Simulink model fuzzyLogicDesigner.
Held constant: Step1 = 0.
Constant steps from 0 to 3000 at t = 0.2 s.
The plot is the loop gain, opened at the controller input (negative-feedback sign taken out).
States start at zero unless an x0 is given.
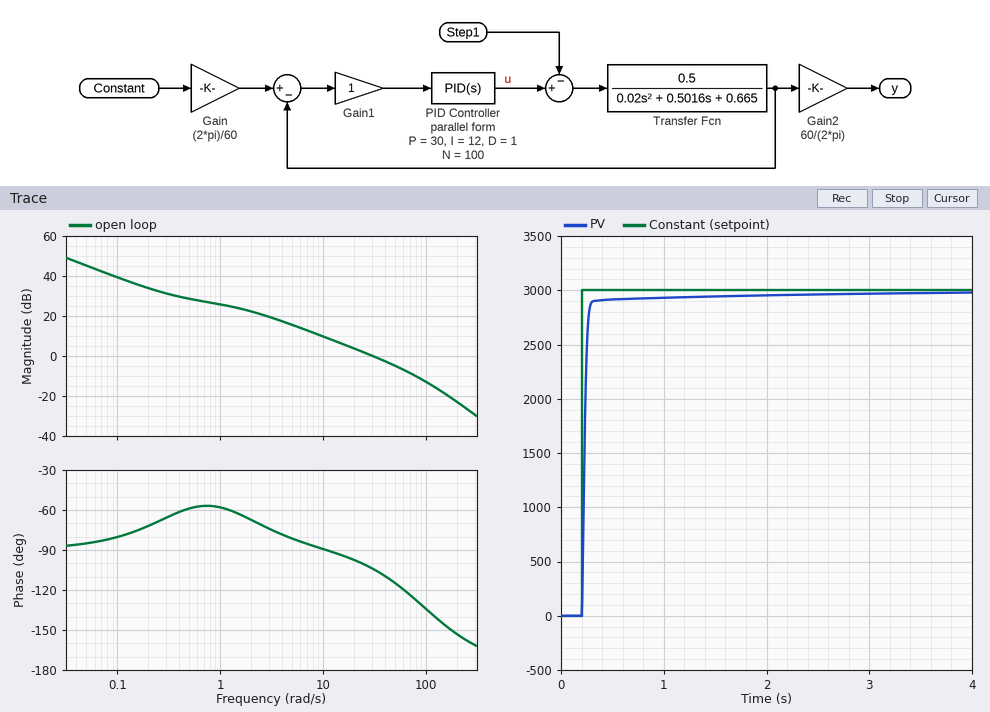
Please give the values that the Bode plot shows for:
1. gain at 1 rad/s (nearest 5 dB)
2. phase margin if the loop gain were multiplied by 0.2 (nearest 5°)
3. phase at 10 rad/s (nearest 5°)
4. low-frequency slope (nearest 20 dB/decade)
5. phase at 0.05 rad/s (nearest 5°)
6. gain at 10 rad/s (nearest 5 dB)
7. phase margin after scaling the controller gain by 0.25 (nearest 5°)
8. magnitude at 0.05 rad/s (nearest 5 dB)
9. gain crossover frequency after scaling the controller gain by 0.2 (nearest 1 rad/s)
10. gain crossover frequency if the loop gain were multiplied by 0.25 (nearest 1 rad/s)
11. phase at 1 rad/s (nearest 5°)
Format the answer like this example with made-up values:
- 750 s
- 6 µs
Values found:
- 25 dB
- 95°
- -90°
- -20 dB/decade
- -85°
- 10 dB
- 95°
- 45 dB
- 6 rad/s
- 8 rad/s
- -60°
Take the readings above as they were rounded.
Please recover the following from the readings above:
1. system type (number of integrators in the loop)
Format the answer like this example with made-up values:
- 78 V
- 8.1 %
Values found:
- 1
